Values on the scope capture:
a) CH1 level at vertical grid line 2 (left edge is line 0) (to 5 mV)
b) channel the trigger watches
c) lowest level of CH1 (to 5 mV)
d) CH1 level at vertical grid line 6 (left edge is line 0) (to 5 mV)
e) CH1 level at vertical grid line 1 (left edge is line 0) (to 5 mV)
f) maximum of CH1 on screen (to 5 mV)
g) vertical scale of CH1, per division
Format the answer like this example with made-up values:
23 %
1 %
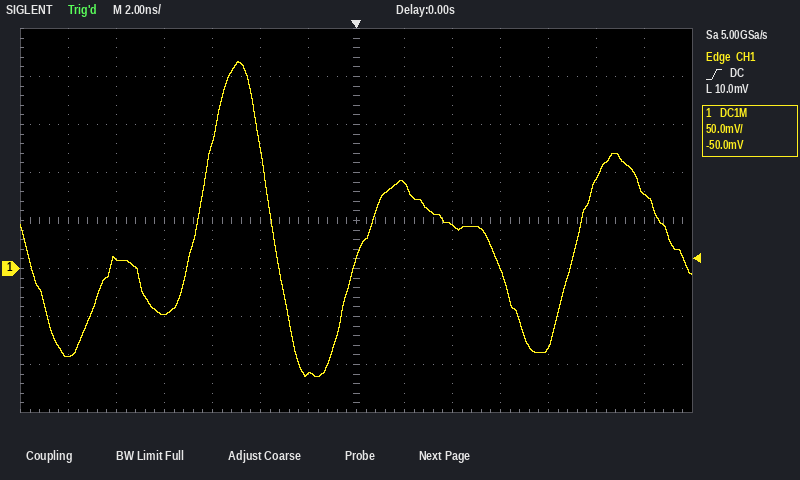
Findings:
10 mV
CH1
-110 mV
-110 mV
-90 mV
215 mV
50 mV
